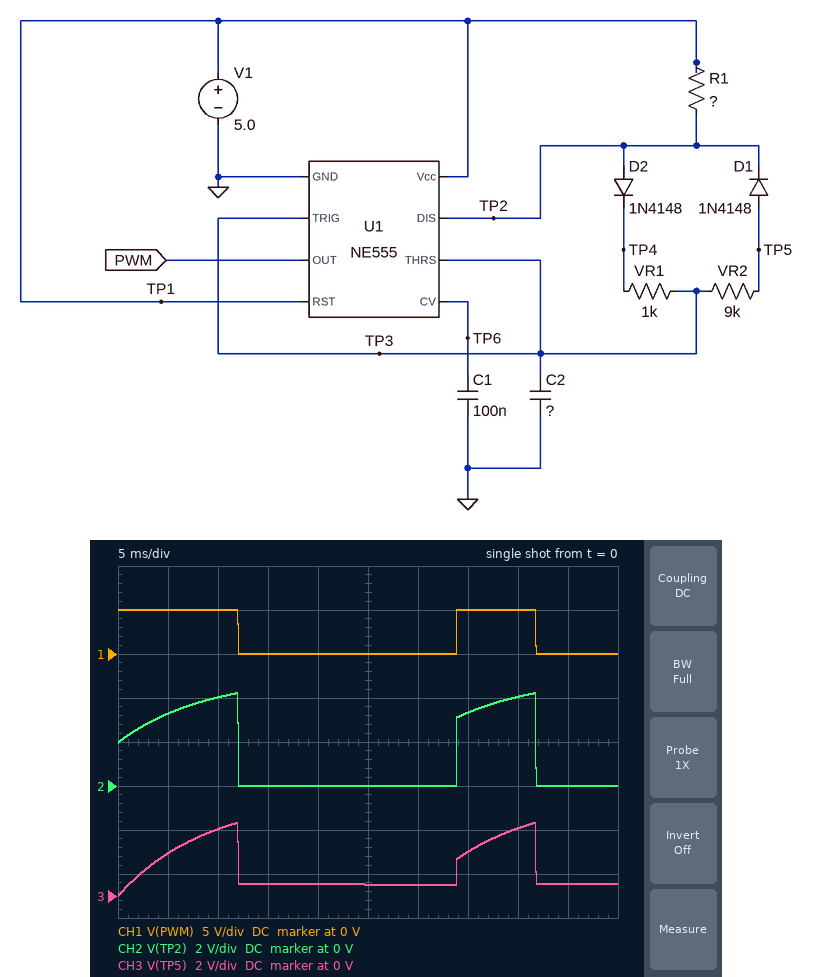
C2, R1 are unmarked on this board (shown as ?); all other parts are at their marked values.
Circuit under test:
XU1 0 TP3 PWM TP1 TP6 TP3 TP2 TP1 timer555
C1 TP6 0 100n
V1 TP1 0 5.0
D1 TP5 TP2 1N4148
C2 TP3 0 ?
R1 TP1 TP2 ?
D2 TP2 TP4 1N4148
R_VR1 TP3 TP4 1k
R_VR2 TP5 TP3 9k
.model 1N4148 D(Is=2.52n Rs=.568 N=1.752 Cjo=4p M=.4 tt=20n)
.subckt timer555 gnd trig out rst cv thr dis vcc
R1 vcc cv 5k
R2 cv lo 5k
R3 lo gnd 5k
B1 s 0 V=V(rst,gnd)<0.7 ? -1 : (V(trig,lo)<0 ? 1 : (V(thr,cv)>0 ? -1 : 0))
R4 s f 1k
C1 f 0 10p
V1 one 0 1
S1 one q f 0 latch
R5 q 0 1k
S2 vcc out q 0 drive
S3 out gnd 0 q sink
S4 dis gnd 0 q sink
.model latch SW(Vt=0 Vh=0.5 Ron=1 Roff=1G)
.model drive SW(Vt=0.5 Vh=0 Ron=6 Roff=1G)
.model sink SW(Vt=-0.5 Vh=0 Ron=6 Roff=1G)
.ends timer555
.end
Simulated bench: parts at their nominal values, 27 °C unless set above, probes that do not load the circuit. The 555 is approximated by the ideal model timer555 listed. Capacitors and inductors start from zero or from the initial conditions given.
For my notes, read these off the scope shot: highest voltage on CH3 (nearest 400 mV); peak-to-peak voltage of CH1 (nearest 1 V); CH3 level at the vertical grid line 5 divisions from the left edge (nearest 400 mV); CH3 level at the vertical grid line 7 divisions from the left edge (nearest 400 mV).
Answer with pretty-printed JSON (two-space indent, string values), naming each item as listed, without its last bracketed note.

{
  "highest voltage on CH3": "3.2 V",
  "peak-to-peak voltage of CH1": "5 V",
  "CH3 level at the vertical grid line 5 divisions from the left edge": "400 mV",
  "CH3 level at the vertical grid line 7 divisions from the left edge": "2.0 V"
}
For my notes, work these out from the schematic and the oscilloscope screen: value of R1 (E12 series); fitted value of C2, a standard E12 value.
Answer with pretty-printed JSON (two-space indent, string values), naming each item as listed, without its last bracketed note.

{
  "value of R1": "2.2 kΩ",
  "fitted value of C2, a standard E12 value": "2.7 µF"
}
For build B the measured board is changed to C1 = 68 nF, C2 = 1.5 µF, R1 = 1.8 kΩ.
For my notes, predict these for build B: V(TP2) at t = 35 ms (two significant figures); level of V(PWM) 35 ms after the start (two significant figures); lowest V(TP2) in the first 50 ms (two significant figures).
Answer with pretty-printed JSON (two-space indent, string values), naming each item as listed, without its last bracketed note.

{
  "V(TP2) at t = 35 ms": "3.6 V",
  "level of V(PWM) 35 ms after the start": "5.0 V",
  "lowest V(TP2) in the first 50 ms": "17 mV"
}
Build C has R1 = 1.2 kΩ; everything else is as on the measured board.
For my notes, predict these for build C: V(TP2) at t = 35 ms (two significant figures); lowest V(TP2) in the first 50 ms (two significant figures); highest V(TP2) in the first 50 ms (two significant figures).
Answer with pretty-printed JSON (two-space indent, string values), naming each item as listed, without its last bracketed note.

{
  "V(TP2) at t = 35 ms": "4.3 V",
  "lowest V(TP2) in the first 50 ms": "26 mV",
  "highest V(TP2) in the first 50 ms": "4.4 V"
}
